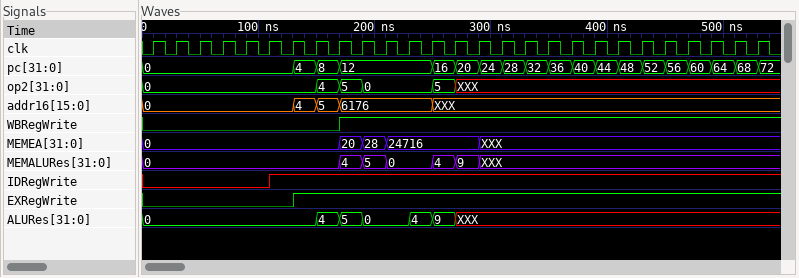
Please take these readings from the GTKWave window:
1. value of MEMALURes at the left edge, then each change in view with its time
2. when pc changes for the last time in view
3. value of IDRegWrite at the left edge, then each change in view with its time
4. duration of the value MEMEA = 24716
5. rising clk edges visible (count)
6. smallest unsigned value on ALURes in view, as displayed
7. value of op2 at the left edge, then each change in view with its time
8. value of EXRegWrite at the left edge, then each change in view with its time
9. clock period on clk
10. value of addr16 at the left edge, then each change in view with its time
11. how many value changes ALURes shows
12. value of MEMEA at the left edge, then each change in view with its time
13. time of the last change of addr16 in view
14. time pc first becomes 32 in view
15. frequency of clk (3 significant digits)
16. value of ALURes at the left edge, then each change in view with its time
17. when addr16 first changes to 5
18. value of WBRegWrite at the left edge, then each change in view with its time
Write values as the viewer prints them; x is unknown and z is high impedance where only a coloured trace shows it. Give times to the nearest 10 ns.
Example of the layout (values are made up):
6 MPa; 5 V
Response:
0, 4 at 170 ns, 5 at 190 ns, 0 at 210 ns, 4 at 250 ns, 9 at 270 ns, XXX at 290 ns; 530 ns; 0, 1 at 110 ns; 80 ns; 27; 0; 0, 4 at 150 ns, 5 at 170 ns, 0 at 190 ns, 5 at 250 ns, XXX at 270 ns; 0, 1 at 130 ns; 20 ns; 0, 4 at 130 ns, 5 at 150 ns, 6176 at 170 ns, XXX at 250 ns; 6; 0, 20 at 170 ns, 28 at 190 ns, 24716 at 210 ns, XXX at 290 ns; 250 ns; 330 ns; 50.0 MHz; 0, 4 at 150 ns, 5 at 170 ns, 0 at 190 ns, 4 at 230 ns, 9 at 250 ns, XXX at 270 ns; 150 ns; 0, 1 at 170 ns
